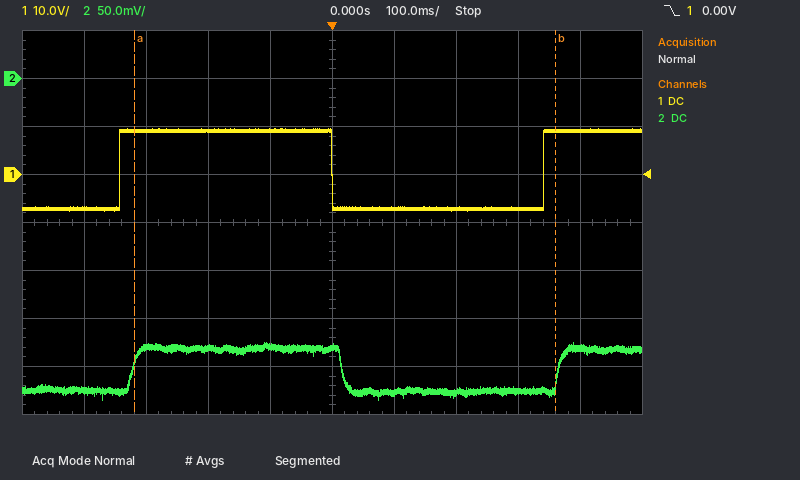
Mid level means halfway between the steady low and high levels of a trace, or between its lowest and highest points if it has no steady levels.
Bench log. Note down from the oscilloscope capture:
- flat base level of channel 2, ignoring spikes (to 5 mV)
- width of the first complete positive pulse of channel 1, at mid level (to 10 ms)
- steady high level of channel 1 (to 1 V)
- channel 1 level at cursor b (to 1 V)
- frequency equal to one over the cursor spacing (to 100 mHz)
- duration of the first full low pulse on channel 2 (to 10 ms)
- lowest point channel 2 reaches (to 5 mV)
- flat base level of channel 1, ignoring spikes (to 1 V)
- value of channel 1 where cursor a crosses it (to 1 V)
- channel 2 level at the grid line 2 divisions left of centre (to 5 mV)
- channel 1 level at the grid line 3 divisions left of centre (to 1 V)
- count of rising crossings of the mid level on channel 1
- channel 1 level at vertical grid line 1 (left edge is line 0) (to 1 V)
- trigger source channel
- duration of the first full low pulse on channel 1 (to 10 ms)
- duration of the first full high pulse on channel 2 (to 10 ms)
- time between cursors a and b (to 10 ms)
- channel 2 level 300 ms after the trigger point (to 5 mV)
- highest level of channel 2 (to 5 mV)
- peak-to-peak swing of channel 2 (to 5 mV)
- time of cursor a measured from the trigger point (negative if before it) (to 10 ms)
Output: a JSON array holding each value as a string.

["-325 mV", "340 ms", "9 V", "9 V", "1.5 Hz", "350 ms", "-335 mV", "-7 V", "9 V", "-280 mV", "9 V", "2", "-7 V", "channel 1", "340 ms", "340 ms", "680 ms", "-325 mV", "-275 mV", "60 mV", "-320 ms"]
